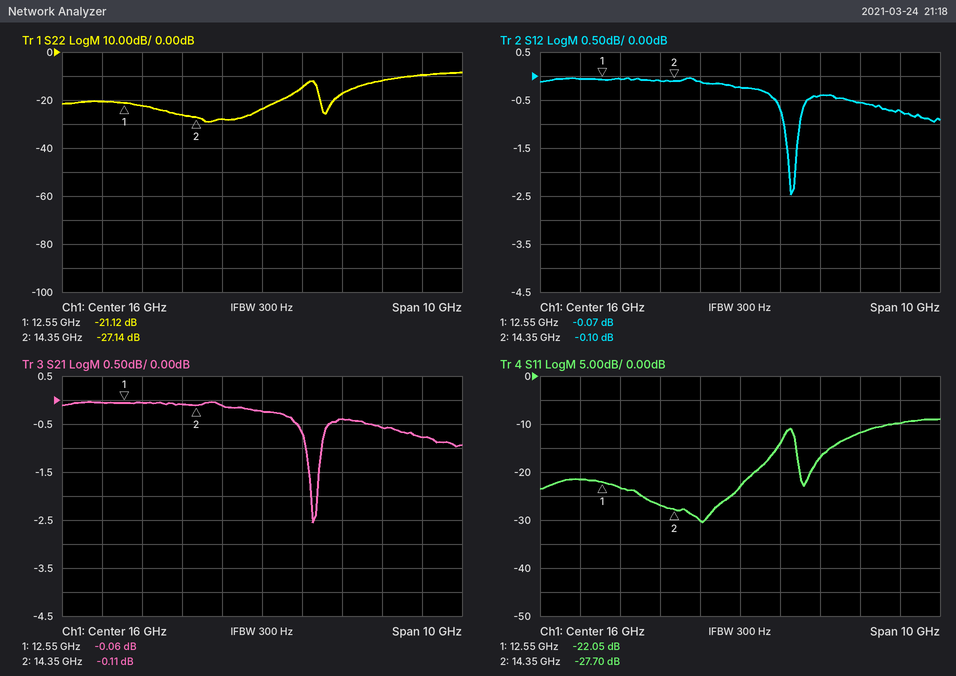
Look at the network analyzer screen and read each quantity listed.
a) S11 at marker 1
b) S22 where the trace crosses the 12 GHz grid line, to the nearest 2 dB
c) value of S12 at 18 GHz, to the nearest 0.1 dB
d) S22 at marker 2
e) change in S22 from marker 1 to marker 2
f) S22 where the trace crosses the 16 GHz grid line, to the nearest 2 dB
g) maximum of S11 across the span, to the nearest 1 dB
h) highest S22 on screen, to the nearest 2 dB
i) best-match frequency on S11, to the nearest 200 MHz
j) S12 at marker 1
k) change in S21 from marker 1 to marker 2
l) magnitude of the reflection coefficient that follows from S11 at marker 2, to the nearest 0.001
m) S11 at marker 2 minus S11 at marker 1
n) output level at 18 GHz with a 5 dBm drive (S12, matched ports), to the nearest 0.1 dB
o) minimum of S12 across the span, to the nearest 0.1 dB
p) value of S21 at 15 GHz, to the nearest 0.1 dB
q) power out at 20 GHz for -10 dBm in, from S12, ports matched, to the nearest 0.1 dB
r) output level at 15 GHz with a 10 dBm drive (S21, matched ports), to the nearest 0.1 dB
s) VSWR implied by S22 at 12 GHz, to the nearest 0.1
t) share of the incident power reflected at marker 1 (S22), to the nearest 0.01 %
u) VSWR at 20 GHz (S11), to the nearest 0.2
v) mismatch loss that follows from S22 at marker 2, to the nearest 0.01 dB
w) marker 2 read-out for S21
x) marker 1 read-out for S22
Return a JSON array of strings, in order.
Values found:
["-22.05 dB", "-20 dB", "-0.4 dB", "-27.14 dB", "-6.02 dB", "-24 dB", "-9 dB", "-8 dB", "15.0 GHz", "-0.07 dB", "-0.05 dB", "0.041", "-5.65 dB", "4.6 dBm", "-2.5 dB", "-0.1 dB", "-10.7 dBm", "9.9 dBm", "1.2", "0.77 %", "2.0", "0.01 dB", "-0.11 dB", "-21.12 dB"]
